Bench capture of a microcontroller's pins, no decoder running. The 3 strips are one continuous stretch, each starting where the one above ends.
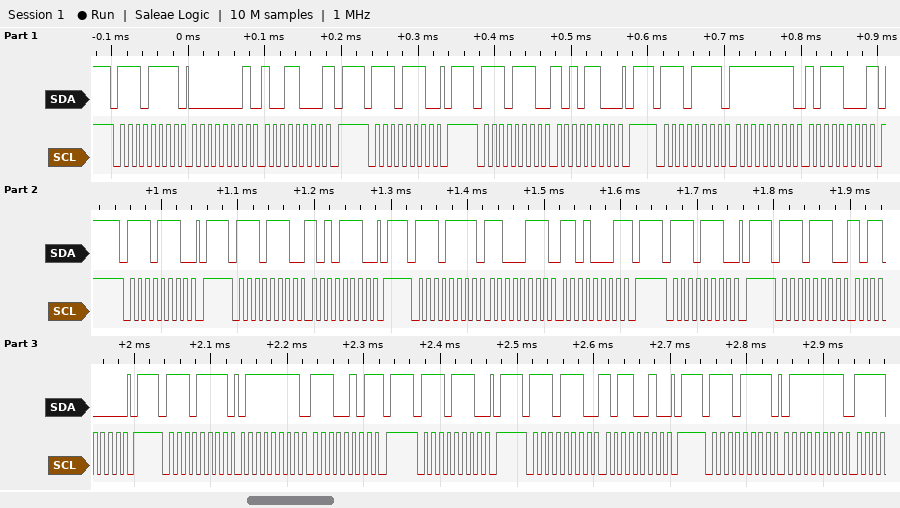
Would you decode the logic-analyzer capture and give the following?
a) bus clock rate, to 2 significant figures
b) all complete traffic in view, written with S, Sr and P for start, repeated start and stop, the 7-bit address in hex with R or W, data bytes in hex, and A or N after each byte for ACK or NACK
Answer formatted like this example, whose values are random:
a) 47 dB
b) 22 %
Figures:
a) 100 kHz
b) S 77R A 01 A 98 N P S 77W A P S 77W A AC A P S 77R A FF A B8 N P S 77W A P S 77W A AE A P S 77R A C7 A D1 N P S 77W A P S 77W A B0 A P S 77R A 7F A E5 N P S 77W A P S 77W A B2 A P S 77R A 7F A
